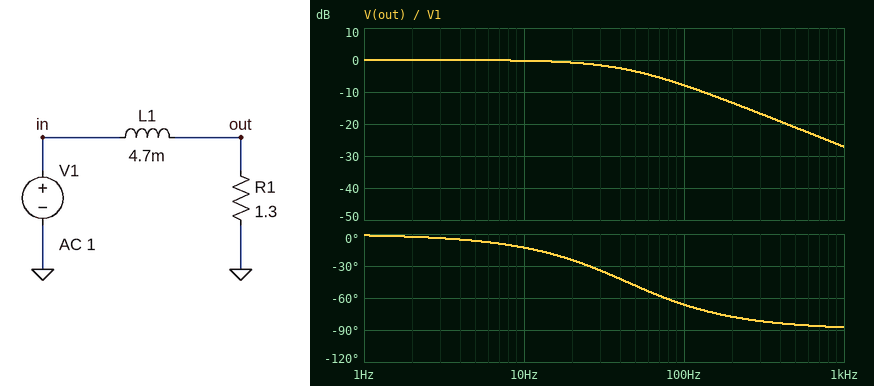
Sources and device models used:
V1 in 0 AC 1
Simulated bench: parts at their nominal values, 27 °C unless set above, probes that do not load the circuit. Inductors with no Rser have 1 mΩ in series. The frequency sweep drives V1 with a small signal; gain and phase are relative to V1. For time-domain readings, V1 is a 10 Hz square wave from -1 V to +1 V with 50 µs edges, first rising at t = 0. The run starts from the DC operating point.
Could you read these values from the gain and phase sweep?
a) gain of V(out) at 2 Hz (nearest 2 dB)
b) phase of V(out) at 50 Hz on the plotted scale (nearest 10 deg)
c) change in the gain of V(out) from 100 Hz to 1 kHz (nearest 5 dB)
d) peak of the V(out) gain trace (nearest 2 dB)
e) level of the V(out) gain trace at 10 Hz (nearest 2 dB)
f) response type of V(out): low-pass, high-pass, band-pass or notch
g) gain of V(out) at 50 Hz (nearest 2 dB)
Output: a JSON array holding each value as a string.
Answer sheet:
["0 dB", "-50 deg", "-20 dB", "0 dB", "0 dB", "low-pass", "-4 dB"]
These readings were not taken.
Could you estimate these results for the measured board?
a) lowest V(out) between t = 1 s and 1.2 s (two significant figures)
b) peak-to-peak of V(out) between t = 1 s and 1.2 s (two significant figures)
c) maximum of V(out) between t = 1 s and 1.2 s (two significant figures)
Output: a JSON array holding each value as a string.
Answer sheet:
["-1.0 V", "2.0 V", "1.0 V"]
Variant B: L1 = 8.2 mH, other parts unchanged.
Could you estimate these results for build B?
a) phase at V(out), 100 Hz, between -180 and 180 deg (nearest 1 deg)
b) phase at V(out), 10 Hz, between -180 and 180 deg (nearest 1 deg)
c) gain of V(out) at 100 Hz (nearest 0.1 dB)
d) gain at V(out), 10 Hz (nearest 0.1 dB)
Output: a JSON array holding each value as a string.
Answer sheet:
["-76 deg", "-22 deg", "-12.2 dB", "-0.6 dB"]
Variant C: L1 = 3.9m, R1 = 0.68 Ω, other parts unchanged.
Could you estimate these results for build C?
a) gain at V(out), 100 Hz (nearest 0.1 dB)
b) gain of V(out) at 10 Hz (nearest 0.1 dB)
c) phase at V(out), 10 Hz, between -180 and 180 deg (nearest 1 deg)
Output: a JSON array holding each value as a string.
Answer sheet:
["-11.5 dB", "-0.5 dB", "-20 deg"]
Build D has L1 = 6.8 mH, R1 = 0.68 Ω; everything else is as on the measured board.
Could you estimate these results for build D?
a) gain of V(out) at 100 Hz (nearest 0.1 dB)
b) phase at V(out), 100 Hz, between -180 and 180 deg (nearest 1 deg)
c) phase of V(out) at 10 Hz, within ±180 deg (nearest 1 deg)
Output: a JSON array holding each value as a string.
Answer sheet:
["-16.1 dB", "-81 deg", "-32 deg"]
